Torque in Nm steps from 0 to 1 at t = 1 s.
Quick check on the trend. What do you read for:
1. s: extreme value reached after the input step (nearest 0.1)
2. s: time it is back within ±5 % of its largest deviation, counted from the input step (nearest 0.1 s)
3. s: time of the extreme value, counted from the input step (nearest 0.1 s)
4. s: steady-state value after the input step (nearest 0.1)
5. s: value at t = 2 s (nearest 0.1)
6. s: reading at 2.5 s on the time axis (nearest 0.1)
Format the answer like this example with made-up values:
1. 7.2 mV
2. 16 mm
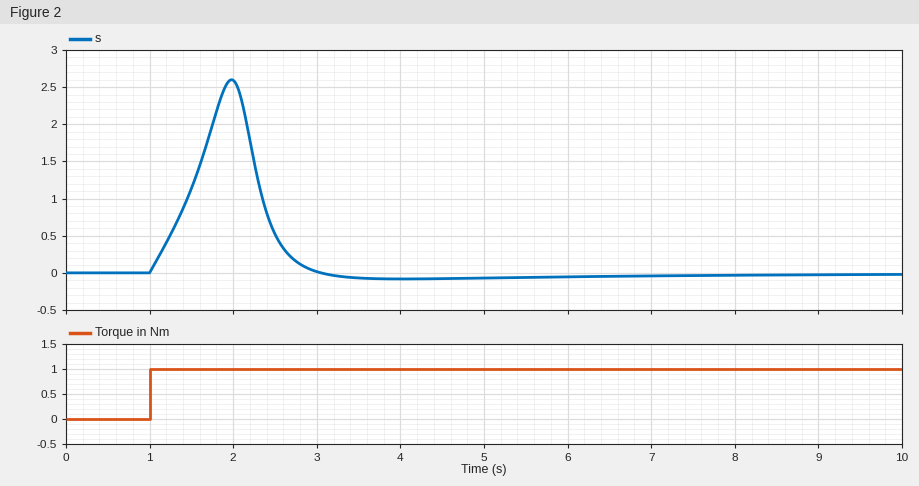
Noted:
1. 2.6
2. 1.8 s
3. 1.0 s
4. 0.0
5. 2.6
6. 0.5
